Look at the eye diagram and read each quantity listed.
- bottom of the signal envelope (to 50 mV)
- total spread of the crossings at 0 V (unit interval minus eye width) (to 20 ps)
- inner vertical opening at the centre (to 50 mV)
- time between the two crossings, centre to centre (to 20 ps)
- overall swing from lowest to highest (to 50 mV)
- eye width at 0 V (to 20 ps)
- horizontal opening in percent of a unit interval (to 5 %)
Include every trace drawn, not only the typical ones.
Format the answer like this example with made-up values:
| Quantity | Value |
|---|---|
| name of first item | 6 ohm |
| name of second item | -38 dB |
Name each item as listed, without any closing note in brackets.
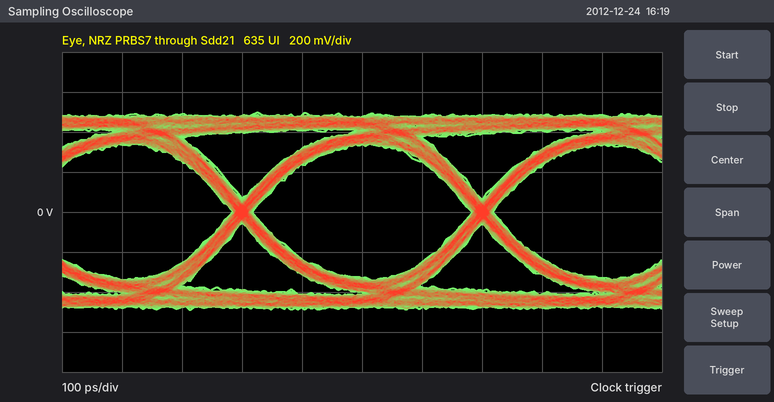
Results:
| Quantity | Value |
|---|---|
| bottom of the signal envelope | -500 mV |
| total spread of the crossings at 0 V (unit interval minus eye width) | 40 ps |
| inner vertical opening at the centre | 650 mV |
| time between the two crossings, centre to centre | 400 ps |
| overall swing from lowest to highest | 1.00 V |
| eye width at 0 V | 360 ps |
| horizontal opening in percent of a unit interval | 90 % |
